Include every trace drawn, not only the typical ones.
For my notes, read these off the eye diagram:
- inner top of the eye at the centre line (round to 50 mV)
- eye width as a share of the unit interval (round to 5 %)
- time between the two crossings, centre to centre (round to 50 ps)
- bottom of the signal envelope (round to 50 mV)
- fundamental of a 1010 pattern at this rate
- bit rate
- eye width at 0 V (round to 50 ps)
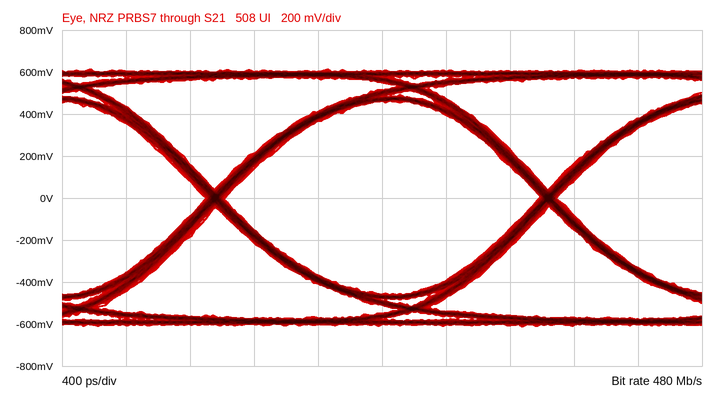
450 mV
95 %
2.10 ns
-600 mV
240 MHz
480 Mb/s
1.95 ns
